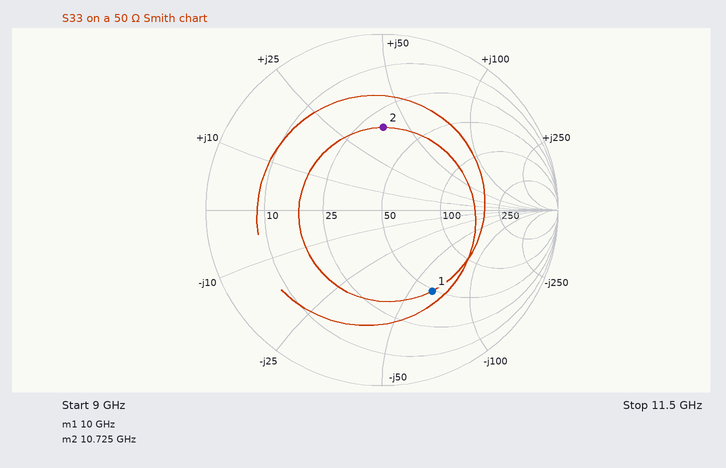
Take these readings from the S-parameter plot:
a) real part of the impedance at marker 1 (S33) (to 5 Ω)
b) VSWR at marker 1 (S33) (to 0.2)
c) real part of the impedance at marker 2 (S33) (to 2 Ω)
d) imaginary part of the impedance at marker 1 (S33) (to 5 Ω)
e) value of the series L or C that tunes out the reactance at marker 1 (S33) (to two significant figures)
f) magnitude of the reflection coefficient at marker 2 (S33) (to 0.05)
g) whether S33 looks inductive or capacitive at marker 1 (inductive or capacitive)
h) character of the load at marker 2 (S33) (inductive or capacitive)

50 Ω
3.4
32 Ω
-65 Ω
1.0 nH
0.45
capacitive
inductive
